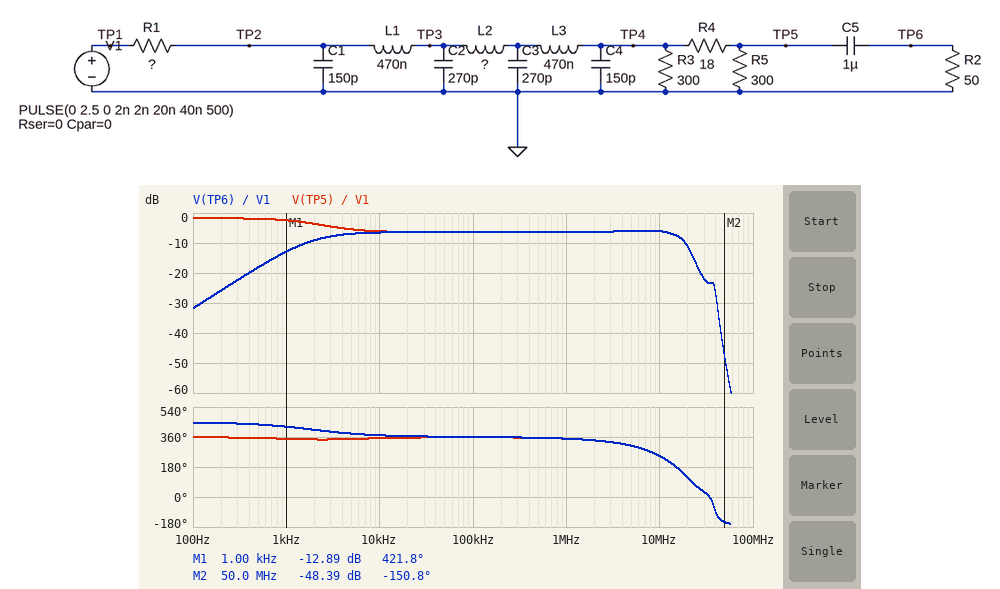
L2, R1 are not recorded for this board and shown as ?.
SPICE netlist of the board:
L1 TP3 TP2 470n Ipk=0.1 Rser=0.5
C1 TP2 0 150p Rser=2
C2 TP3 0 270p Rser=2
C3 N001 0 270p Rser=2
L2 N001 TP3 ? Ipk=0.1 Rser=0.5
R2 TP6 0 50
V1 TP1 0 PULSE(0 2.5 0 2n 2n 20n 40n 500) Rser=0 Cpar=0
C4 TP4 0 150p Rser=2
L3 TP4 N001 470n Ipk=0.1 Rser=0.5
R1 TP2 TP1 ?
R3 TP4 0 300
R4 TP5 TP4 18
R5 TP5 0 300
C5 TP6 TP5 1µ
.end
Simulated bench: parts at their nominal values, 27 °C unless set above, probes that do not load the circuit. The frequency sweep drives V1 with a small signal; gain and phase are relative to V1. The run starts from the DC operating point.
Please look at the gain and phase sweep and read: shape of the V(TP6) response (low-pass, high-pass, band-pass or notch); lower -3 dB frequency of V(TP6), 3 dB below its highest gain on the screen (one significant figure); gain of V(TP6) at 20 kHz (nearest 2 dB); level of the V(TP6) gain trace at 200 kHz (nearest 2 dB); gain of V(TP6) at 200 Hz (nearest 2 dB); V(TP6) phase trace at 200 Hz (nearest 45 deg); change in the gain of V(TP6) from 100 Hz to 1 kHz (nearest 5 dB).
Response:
band-pass
2 kHz
-6 dB
-6 dB
-26 dB
450 deg
20 dB
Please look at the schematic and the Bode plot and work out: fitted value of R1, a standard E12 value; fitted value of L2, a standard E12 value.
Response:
22 Ω
150 nH
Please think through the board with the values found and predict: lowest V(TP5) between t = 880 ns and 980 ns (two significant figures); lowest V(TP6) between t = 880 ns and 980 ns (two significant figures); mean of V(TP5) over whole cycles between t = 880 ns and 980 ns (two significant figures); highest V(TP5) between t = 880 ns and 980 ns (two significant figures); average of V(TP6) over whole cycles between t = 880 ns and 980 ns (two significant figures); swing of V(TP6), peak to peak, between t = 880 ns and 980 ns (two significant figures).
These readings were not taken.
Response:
450 mV
440 mV
670 mV
880 mV
650 mV
420 mV
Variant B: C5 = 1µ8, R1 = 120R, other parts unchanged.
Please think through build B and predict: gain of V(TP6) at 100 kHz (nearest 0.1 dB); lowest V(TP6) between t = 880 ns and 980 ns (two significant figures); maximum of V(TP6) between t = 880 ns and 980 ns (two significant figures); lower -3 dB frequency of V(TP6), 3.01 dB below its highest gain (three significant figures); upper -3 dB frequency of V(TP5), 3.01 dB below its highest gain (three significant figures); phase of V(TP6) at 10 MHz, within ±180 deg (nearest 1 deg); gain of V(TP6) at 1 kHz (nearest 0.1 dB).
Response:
-13.7 dB
150 mV
420 mV
693 Hz
833 Hz
-108 deg
-15.4 dB
